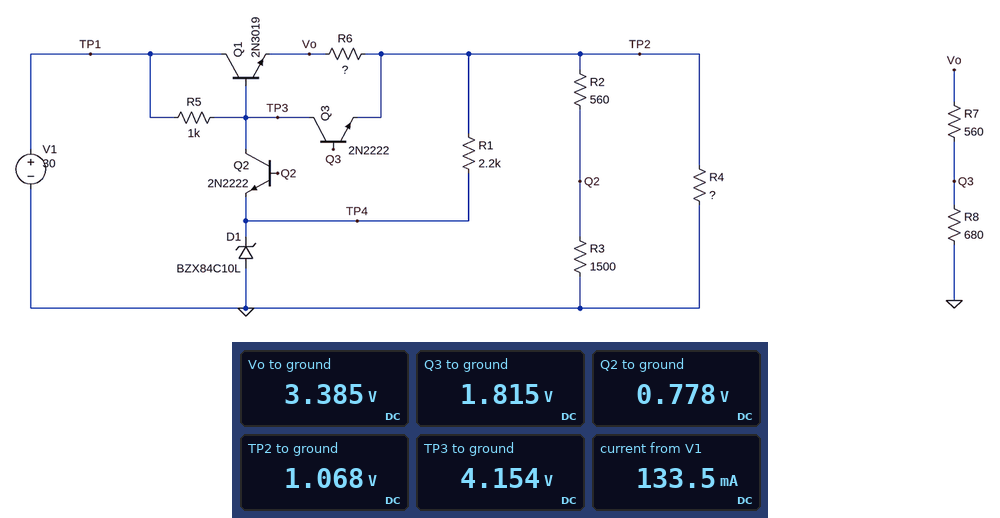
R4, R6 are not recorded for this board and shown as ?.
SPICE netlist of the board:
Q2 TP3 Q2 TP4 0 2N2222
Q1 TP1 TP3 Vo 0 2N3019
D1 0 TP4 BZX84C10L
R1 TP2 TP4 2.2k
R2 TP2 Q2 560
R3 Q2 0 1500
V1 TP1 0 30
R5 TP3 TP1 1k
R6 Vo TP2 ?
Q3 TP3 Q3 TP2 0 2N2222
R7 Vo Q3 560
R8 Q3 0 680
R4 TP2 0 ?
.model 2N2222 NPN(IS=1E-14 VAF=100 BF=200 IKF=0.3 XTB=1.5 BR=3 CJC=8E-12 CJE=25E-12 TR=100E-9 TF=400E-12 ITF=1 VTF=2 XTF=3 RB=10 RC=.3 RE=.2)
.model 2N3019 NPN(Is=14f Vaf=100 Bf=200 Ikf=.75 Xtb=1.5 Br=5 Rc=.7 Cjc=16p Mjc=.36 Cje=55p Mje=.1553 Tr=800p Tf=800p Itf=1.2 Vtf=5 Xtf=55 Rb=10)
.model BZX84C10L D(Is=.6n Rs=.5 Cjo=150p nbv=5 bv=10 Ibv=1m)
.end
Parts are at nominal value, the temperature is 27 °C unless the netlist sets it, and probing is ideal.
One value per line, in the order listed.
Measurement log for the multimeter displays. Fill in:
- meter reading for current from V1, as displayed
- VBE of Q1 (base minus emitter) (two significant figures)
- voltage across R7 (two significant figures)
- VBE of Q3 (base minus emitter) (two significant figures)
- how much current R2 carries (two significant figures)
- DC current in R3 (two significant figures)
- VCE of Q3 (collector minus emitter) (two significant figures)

133.5 mA
770 mV
1.6 V
750 mV
520 µA
520 µA
3.1 V
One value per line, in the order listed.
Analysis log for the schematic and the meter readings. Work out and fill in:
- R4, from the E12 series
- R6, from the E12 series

8.2 Ω
22 Ω
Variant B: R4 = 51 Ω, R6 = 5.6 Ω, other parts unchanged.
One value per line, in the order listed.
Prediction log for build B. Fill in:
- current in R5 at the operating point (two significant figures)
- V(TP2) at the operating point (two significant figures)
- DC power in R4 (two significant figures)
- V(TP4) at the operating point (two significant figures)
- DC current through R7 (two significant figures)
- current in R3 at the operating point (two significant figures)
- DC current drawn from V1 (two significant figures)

12 mA
15 V
4.5 W
10 V
14 mA
7.4 mA
330 mA
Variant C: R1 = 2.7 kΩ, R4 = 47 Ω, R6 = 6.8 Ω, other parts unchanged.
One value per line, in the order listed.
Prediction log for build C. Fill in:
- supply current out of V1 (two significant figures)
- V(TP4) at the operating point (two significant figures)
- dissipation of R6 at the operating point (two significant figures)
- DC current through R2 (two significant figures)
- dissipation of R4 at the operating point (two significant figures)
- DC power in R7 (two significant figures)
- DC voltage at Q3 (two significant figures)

360 mA
10 V
750 mW
7.4 mA
4.9 W
110 mW
9.6 V
